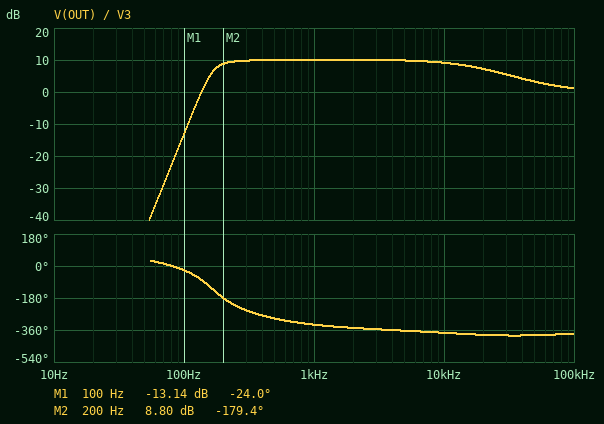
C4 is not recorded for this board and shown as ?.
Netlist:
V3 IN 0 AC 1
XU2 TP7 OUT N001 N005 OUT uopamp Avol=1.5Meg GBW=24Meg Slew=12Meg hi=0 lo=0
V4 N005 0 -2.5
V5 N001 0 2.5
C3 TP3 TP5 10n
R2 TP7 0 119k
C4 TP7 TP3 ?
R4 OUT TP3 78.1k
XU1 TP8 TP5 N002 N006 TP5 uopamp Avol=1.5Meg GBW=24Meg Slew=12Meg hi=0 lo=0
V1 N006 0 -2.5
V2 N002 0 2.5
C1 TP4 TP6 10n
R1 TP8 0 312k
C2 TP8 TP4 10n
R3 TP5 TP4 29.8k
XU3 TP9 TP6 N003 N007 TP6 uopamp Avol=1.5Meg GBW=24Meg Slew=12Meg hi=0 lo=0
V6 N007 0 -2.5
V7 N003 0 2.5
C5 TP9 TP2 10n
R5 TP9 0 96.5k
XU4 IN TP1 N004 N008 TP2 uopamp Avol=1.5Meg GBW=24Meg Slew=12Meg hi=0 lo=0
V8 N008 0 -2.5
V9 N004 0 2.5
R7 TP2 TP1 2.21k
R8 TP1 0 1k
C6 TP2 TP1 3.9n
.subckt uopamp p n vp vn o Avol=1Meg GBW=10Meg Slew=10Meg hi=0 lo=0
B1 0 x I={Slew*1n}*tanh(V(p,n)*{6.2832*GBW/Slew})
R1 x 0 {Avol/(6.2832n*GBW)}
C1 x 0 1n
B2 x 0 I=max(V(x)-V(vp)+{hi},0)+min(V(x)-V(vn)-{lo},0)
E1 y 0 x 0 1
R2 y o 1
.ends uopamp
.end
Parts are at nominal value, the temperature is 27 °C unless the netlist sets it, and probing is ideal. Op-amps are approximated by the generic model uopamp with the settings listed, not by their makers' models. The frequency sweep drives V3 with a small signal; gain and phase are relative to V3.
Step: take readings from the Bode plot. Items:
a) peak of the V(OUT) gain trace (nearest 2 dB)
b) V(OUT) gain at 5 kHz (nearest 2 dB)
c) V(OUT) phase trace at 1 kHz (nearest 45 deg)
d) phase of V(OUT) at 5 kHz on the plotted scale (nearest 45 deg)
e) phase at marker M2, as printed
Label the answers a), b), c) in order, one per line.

a) 10 dB
b) 10 dB
c) -315 deg
d) -360 deg
e) -179.4 deg
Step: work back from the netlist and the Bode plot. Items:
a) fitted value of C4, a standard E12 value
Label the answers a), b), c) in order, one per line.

a) 8.2 nF
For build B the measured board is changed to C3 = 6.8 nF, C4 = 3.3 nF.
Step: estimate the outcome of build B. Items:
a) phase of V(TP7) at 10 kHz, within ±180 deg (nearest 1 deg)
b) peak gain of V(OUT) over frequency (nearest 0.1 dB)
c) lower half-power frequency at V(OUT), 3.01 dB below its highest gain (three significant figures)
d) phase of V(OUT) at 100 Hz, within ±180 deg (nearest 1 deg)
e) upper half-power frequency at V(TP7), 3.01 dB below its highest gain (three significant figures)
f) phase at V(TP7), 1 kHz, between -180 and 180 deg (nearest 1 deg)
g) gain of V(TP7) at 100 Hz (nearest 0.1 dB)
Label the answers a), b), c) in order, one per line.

a) -14 deg
b) 10.0 dB
c) 397 Hz
d) 0 deg
e) 21.3 kHz
f) 48 deg
g) -23.7 dB
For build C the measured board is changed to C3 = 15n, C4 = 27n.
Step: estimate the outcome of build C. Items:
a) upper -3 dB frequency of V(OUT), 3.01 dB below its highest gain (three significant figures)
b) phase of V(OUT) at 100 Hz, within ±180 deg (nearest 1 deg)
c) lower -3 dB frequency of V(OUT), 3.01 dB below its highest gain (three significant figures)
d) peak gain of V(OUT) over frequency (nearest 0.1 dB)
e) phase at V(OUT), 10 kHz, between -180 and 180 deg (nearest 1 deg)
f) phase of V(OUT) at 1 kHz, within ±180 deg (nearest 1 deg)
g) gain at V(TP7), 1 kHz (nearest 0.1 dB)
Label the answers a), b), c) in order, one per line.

a) 12.9 kHz
b) -75 deg
c) 152 Hz
d) 11.6 dB
e) -17 deg
f) 21 deg
g) 10.2 dB
